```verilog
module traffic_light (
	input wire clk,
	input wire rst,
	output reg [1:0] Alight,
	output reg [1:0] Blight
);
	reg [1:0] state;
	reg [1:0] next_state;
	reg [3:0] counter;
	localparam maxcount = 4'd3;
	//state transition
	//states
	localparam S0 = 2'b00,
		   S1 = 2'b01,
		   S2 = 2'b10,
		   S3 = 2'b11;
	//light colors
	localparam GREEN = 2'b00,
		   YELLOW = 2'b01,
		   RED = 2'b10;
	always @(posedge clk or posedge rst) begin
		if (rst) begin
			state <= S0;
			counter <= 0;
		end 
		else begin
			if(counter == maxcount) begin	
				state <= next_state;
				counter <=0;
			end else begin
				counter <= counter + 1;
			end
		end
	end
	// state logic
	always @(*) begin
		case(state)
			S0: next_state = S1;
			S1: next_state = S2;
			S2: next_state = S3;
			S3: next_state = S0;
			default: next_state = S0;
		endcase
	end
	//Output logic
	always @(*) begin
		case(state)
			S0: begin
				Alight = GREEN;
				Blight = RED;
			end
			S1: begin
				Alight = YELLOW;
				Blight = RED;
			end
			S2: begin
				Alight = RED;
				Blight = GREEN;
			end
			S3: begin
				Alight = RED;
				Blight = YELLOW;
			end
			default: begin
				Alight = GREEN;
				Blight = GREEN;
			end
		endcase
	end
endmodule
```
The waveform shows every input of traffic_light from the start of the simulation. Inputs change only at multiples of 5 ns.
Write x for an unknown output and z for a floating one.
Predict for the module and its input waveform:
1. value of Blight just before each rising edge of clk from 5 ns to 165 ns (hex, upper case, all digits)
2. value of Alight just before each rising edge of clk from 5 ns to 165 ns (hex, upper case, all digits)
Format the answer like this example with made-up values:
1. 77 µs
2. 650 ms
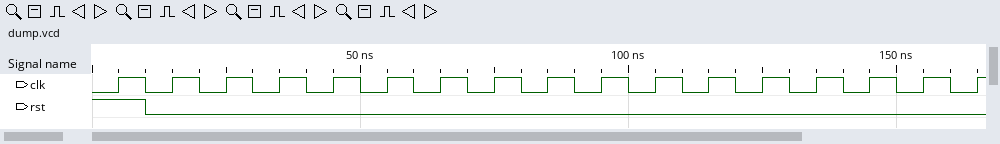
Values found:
1. 2, 2, 2, 2, 2, 2, 2, 2, 2, 0, 0, 0, 0, 1, 1, 1, 1
2. 0, 0, 0, 0, 0, 1, 1, 1, 1, 2, 2, 2, 2, 2, 2, 2, 2
